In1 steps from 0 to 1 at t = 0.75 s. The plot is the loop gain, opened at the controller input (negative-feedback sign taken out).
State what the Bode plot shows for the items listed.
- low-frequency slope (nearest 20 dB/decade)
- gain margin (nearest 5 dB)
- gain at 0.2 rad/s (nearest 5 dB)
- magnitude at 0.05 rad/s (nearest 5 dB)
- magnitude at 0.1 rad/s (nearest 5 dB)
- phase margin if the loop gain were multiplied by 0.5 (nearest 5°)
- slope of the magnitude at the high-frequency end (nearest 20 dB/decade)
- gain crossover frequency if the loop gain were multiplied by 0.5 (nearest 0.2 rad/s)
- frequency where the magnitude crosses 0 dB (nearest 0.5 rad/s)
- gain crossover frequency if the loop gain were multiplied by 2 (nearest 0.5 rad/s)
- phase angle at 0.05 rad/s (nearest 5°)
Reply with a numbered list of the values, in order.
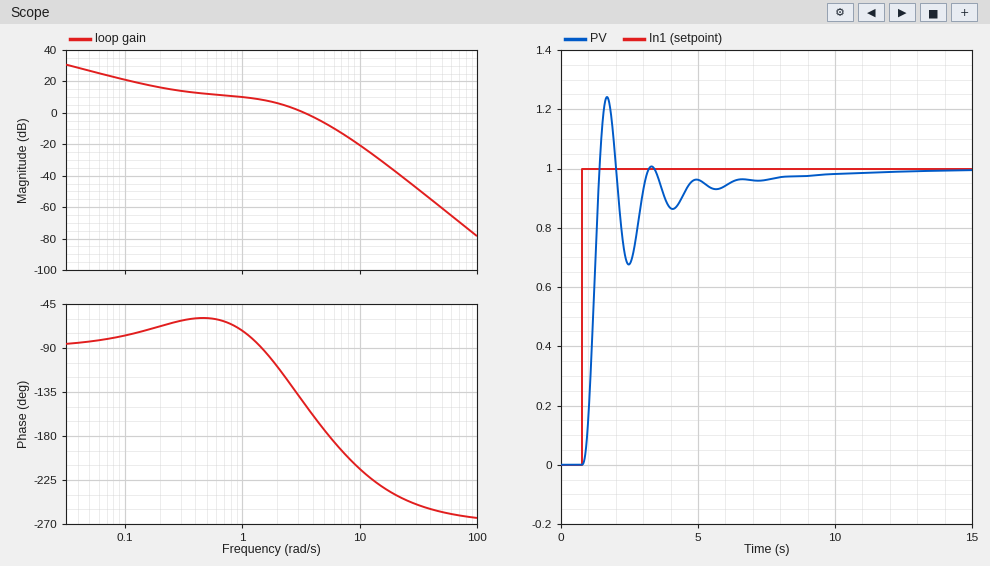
1. -20 dB/decade
2. 10 dB
3. 15 dB
4. 25 dB
5. 20 dB
6. 70°
7. -60 dB/decade
8. 2.0 rad/s
9. 3.5 rad/s
10. 5.0 rad/s
11. -85°
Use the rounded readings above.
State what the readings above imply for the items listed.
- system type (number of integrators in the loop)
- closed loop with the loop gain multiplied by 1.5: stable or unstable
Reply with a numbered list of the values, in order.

1. 1
2. stable
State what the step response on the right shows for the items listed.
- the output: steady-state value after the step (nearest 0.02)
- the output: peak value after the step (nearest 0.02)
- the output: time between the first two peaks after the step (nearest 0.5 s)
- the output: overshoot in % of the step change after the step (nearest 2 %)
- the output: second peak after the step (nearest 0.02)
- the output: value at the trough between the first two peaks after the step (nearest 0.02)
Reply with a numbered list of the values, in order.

1. 1.00
2. 1.24
3. 1.5 s
4. 24 %
5. 1.00
6. 0.68
